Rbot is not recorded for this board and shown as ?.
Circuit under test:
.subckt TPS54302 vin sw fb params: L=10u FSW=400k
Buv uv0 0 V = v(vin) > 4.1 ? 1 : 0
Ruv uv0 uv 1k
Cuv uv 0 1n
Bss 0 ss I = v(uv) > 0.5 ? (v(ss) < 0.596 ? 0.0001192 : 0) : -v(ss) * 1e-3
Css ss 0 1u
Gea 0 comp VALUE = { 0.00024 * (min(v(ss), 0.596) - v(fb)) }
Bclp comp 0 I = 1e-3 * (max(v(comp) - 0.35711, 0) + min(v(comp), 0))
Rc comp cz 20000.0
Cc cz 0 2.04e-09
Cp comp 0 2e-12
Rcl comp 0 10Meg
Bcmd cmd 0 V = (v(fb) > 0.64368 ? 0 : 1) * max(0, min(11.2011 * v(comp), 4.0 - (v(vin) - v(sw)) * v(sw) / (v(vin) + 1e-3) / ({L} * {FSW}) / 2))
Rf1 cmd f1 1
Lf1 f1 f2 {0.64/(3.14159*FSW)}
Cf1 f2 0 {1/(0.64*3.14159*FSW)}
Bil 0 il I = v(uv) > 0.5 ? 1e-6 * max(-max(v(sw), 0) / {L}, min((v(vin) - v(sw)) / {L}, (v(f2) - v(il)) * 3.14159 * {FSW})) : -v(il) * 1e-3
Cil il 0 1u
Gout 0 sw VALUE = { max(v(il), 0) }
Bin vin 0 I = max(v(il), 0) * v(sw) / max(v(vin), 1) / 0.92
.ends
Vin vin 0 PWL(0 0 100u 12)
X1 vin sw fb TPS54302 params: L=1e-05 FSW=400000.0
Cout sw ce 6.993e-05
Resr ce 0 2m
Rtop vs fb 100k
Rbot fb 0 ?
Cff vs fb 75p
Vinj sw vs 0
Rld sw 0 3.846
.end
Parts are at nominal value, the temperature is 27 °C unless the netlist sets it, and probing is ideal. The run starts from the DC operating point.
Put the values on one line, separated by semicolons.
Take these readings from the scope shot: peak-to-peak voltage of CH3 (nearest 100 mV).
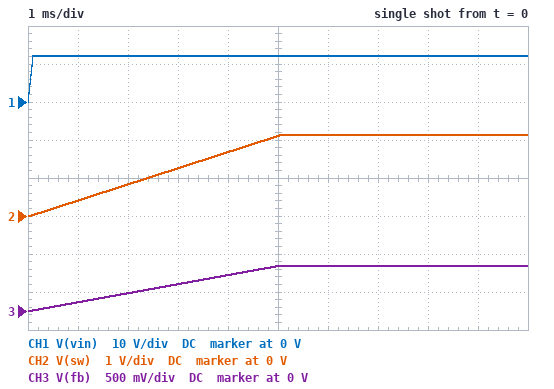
600 mV
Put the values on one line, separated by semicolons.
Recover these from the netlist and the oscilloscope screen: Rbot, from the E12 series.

39 kΩ
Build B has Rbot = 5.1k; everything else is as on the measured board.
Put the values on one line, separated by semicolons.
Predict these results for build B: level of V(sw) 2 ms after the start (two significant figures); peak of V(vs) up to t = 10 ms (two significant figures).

4.8 V; 12 V
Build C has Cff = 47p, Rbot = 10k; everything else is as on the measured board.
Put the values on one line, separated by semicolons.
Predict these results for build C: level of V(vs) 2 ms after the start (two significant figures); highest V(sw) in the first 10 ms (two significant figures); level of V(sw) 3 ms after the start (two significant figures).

2.6 V; 6.6 V; 3.9 V
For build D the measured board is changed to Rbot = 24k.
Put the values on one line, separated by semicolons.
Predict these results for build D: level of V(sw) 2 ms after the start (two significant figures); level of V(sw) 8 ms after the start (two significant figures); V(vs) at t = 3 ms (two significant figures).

1.2 V; 3.1 V; 1.8 V
